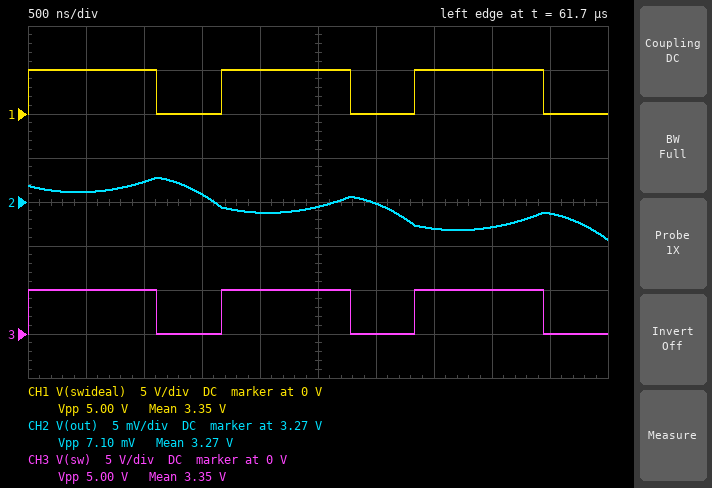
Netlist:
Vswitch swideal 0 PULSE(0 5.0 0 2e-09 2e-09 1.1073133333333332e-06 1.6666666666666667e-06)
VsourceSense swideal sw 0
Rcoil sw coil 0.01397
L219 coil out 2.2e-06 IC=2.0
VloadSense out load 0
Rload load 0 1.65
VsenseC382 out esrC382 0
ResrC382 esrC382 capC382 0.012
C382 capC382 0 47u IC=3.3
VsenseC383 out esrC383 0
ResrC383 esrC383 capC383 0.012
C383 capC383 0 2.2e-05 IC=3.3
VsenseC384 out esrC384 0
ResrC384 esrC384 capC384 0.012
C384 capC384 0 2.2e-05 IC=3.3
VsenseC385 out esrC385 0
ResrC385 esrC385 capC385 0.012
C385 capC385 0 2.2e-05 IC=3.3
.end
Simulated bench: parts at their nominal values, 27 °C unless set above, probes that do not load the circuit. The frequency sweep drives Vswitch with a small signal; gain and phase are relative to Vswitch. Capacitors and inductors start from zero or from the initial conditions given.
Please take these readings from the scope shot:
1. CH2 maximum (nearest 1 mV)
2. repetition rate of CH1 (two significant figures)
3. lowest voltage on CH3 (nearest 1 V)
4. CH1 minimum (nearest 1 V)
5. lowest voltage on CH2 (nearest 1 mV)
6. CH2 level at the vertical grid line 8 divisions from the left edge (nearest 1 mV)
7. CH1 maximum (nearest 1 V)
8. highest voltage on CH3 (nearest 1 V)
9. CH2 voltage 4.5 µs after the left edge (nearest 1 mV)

3.273 V
600 kHz
0 V
0 V
3.266 V
3.267 V
5 V
5 V
3.269 V
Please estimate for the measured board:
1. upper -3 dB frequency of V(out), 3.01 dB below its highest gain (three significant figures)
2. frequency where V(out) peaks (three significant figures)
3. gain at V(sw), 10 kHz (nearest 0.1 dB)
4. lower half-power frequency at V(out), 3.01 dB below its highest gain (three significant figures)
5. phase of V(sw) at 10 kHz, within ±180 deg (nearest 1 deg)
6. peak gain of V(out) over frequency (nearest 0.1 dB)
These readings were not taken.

11.0 kHz
10.0 kHz
0 dB
8.89 kHz
0 deg
13.6 dB
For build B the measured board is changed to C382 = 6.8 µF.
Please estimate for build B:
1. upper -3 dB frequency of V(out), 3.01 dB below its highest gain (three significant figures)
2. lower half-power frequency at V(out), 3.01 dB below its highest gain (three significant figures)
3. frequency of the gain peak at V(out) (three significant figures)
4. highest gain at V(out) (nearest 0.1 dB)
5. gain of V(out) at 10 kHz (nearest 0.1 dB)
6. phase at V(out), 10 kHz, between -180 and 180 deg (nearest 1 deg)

13.7 kHz
11.1 kHz
12.5 kHz
13.8 dB
7.8 dB
-23 deg
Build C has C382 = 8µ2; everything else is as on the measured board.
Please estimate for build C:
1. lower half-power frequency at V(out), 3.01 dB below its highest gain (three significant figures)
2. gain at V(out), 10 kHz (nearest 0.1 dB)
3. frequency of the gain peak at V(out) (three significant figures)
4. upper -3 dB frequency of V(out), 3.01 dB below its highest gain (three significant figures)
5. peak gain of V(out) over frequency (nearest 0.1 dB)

11.0 kHz
8.0 dB
12.4 kHz
13.6 kHz
13.8 dB
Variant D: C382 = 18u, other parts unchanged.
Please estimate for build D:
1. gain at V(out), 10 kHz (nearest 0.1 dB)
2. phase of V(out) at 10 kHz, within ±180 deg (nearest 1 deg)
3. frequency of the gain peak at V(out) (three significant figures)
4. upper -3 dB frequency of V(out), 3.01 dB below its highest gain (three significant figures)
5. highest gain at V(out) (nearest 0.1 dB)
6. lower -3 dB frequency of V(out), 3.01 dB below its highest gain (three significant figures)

9.7 dB
-31 deg
11.6 kHz
12.8 kHz
13.9 dB
10.4 kHz
